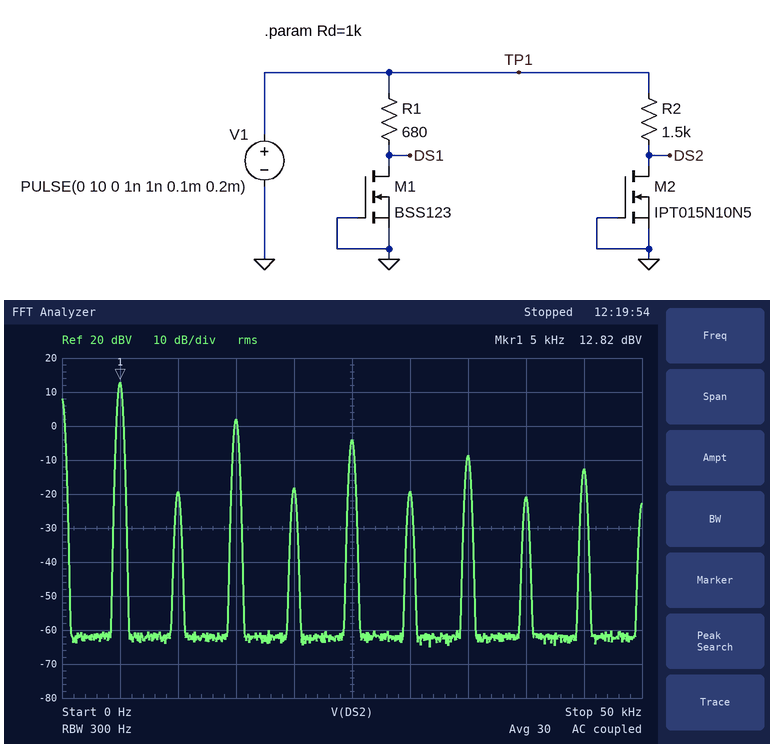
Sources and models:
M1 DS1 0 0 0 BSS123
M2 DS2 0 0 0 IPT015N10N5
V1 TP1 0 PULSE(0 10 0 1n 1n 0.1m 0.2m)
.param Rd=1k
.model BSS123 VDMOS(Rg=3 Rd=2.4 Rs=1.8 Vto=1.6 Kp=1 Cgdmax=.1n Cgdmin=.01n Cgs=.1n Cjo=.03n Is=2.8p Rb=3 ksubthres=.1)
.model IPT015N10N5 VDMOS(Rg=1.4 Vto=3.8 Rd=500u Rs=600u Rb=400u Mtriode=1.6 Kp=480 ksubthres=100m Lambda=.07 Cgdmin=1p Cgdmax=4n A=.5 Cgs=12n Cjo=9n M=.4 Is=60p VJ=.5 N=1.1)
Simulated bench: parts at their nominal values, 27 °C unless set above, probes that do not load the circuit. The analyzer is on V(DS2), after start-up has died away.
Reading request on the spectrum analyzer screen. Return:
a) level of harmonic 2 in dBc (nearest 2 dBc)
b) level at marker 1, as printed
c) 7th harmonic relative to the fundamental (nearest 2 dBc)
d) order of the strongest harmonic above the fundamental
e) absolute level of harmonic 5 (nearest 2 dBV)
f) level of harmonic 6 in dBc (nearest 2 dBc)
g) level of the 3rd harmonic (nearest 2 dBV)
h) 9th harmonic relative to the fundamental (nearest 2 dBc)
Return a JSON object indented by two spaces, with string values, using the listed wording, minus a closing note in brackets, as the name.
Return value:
{
  "level of harmonic 2 in dBc": "-32 dBc",
  "level at marker 1, as printed": "12.82 dBV",
  "7th harmonic relative to the fundamental": "-22 dBc",
  "order of the strongest harmonic above the fundamental": "3",
  "absolute level of harmonic 5": "-4 dBV",
  "level of harmonic 6 in dBc": "-32 dBc",
  "level of the 3rd harmonic": "2 dBV",
  "9th harmonic relative to the fundamental": "-26 dBc"
}
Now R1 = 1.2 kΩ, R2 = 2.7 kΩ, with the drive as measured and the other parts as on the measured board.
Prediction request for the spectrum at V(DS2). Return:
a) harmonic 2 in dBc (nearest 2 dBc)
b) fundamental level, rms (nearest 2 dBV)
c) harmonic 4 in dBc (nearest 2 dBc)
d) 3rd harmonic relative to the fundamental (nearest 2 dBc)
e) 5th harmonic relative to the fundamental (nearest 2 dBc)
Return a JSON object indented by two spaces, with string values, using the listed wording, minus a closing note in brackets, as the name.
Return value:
{
  "harmonic 2 in dBc": "-26 dBc",
  "fundamental level, rms": "12 dBV",
  "harmonic 4 in dBc": "-28 dBc",
  "3rd harmonic relative to the fundamental": "-12 dBc",
  "5th harmonic relative to the fundamental": "-20 dBc"
}
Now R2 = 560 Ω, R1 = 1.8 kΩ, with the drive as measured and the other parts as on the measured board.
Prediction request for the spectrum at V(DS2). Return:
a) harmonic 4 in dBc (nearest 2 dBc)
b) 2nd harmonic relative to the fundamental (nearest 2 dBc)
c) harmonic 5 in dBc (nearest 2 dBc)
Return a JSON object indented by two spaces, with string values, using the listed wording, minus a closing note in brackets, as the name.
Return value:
{
  "harmonic 4 in dBc": "-42 dBc",
  "2nd harmonic relative to the fundamental": "-46 dBc",
  "harmonic 5 in dBc": "-14 dBc"
}
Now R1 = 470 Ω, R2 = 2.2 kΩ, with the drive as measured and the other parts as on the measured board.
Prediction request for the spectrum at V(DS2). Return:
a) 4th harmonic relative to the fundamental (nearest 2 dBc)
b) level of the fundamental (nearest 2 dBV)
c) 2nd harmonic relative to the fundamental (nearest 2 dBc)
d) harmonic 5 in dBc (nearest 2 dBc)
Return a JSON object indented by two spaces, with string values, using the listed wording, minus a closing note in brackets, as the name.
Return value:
{
  "4th harmonic relative to the fundamental": "-28 dBc",
  "level of the fundamental": "12 dBV",
  "2nd harmonic relative to the fundamental": "-28 dBc",
  "harmonic 5 in dBc": "-18 dBc"
}
